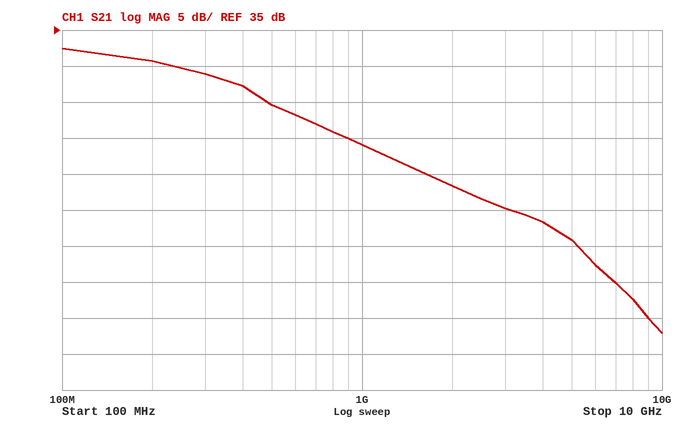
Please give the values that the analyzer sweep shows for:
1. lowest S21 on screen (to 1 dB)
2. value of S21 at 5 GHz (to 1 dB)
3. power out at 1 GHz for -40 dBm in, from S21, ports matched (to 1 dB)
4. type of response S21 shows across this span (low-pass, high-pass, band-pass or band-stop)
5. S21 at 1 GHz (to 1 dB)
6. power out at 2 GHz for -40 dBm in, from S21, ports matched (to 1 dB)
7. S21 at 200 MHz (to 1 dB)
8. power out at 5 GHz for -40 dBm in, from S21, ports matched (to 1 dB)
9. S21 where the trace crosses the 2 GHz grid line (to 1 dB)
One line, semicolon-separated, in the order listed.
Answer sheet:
-7 dB; 6 dB; -21 dBm; low-pass; 19 dB; -27 dBm; 31 dB; -34 dBm; 13 dB
